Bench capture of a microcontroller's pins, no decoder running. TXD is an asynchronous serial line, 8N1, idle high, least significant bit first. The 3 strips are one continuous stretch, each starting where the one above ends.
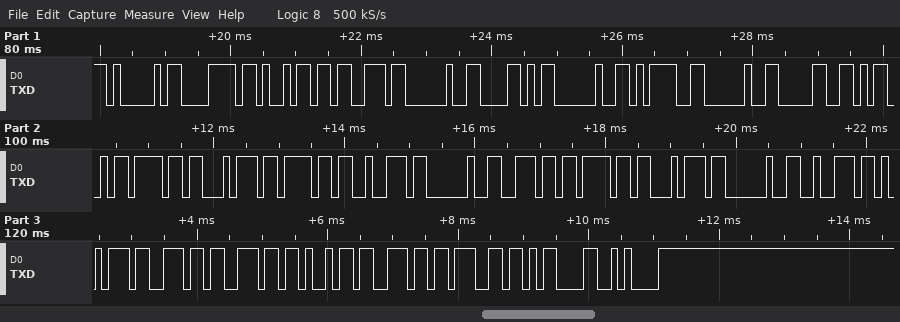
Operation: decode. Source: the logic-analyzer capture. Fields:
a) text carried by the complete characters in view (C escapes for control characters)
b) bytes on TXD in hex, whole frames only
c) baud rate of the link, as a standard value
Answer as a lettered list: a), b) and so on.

a) "Axis X = 0Motor not running\r\n"
b) 0x41 0x78 0x69 0x73 0x20 0x58 0x20 0x3D 0x20 0x30 0x4D 0x6F 0x74 0x6F 0x72 0x20 0x6E 0x6F 0x74 0x20 0x72 0x75 0x6E 0x6E 0x69 0x6E 0x67 0x0D 0x0A
c) 9600 baud
